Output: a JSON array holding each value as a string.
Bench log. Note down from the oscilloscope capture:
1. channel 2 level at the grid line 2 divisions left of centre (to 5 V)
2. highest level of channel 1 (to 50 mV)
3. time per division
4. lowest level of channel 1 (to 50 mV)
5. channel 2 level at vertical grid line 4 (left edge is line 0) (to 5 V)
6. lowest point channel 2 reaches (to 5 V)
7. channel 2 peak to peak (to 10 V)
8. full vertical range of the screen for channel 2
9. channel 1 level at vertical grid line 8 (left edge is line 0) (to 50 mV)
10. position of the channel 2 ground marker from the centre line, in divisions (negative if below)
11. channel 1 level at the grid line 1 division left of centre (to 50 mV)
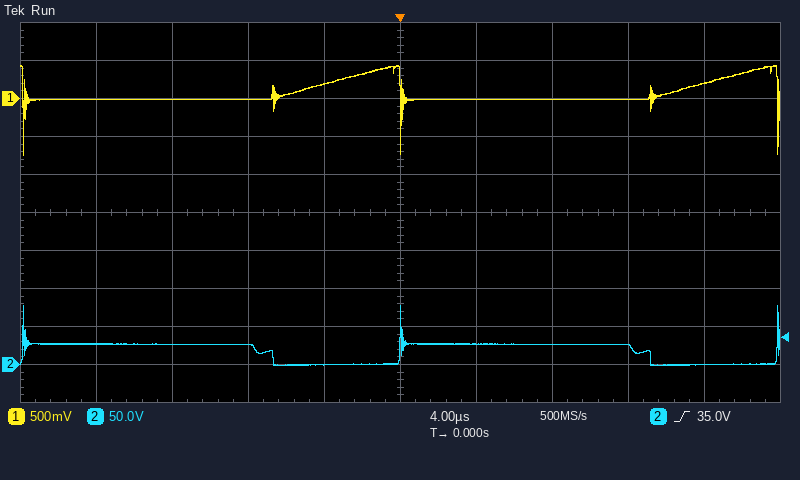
["25 V", "450 mV", "4 µs", "-750 mV", "0 V", "0 V", "80 V", "500 V", "0 mV", "-4.0 div", "200 mV"]
